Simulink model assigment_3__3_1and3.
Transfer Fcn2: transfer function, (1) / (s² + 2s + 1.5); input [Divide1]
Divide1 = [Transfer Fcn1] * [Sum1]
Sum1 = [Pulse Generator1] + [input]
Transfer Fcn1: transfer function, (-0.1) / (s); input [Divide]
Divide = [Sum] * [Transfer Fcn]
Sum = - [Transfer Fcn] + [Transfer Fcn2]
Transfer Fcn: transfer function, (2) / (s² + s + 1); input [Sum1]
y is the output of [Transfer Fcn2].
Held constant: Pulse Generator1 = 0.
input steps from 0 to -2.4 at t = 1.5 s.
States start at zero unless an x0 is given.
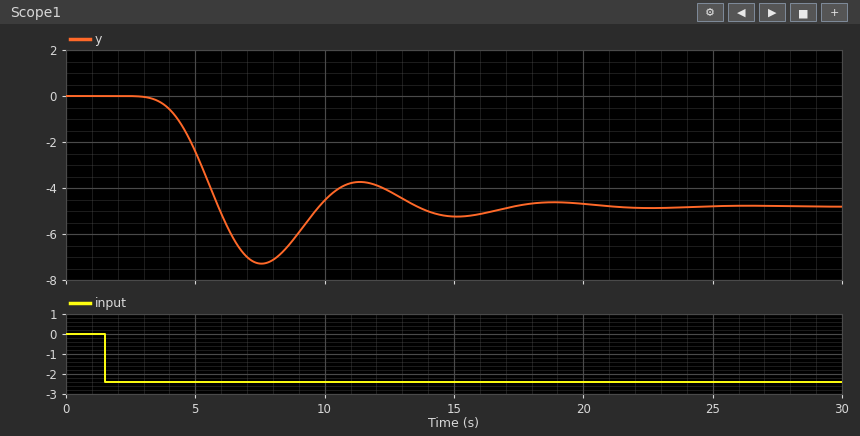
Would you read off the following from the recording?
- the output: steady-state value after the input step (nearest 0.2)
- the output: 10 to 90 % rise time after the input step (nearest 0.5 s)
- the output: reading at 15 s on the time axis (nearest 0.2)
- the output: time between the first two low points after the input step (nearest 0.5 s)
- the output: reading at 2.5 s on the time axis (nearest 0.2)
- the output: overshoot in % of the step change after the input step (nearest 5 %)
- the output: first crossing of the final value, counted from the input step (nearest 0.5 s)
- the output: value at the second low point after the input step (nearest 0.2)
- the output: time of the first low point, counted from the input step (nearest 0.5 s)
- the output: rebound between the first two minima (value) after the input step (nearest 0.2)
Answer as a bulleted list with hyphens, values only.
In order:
- -4.8
- 2.0 s
- -5.2
- 7.5 s
- 0.0
- 50 %
- 4.5 s
- -5.2
- 6.0 s
- -3.8
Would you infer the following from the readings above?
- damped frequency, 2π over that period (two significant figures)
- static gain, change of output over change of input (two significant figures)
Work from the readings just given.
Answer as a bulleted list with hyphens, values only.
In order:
- 0.84 rad/s
- 2.0
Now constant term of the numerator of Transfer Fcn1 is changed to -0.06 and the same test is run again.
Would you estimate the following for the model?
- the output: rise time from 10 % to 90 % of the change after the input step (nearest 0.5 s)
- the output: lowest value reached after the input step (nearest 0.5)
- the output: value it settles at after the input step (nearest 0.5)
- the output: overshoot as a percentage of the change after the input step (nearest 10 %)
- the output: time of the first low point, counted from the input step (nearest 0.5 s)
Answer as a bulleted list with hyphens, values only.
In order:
- 2.5 s
- -6.0
- -5.0
- 30 %
- 7.0 s
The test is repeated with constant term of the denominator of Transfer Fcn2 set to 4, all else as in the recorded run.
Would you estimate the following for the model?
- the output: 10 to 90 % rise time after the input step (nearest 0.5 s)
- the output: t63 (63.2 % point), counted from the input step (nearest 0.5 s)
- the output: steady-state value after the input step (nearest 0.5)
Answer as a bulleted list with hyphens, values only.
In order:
- 5.0 s
- 4.5 s
- -5.0
